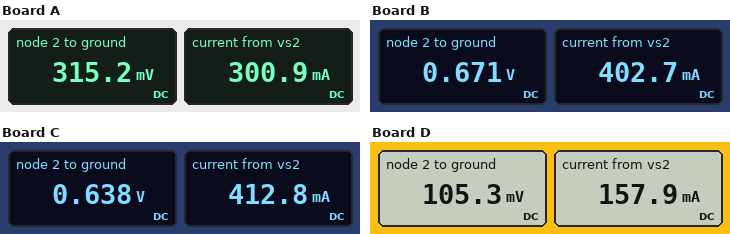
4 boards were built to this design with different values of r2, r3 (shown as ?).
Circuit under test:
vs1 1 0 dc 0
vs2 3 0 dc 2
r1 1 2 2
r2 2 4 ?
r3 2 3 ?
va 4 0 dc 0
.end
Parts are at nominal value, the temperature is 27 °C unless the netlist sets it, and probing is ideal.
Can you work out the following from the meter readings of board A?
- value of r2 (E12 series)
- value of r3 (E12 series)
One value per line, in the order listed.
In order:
2.2 Ω
5.6 Ω
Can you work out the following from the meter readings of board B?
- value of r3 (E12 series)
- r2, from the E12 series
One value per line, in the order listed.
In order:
3.3 Ω
10 Ω
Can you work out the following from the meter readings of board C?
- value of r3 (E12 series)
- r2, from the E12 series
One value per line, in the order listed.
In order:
3.3 Ω
6.8 Ω
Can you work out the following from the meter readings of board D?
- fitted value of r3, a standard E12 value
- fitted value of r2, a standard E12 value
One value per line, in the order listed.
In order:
12 Ω
1 Ω
